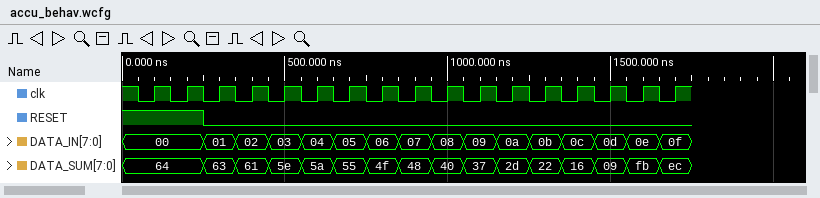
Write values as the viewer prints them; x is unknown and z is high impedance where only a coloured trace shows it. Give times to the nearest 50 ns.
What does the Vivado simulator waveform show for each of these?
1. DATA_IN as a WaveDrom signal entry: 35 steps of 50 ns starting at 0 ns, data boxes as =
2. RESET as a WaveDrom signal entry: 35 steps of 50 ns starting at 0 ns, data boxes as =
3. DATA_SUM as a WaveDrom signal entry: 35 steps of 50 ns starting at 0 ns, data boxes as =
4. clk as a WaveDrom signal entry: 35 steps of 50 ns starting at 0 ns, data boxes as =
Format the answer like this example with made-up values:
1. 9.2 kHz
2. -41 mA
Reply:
1. {name: 'DATA_IN', wave: '=....=.=.=.=.=.=.=.=.=.=.=.=.=.=.=.', data: '00 01 02 03 04 05 06 07 08 09 0a 0b 0c 0d 0e 0f'}
2. {name: 'RESET', wave: '1....0.............................'}
3. {name: 'DATA_SUM', wave: '=....=.=.=.=.=.=.=.=.=.=.=.=.=.=.=.', data: '64 63 61 5e 5a 55 4f 48 40 37 2d 22 16 09 fb ec'}
4. {name: 'clk', wave: '10101010101010101010101010101010101'}
